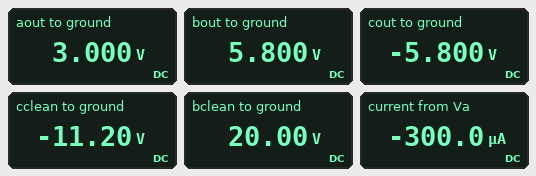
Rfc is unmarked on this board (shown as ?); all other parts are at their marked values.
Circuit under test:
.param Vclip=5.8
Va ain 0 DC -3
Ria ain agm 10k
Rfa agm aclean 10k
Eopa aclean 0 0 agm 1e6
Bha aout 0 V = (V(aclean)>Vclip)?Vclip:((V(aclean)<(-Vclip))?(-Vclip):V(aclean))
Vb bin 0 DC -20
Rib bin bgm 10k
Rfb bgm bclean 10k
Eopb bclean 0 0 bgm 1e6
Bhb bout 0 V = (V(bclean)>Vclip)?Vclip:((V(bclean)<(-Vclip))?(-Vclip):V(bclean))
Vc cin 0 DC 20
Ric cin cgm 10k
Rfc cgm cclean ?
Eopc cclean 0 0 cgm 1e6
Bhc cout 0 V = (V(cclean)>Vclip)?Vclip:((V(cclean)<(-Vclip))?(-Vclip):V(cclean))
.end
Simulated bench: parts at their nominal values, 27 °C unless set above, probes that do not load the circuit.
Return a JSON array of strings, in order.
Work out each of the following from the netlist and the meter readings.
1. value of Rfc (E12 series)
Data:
["5.6 kΩ"]
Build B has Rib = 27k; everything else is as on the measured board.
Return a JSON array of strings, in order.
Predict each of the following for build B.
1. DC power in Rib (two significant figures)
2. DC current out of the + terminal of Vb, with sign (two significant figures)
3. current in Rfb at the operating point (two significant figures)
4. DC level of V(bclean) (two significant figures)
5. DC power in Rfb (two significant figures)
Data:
["15 mW", "-740 µA", "740 µA", "7.4 V", "5.5 mW"]
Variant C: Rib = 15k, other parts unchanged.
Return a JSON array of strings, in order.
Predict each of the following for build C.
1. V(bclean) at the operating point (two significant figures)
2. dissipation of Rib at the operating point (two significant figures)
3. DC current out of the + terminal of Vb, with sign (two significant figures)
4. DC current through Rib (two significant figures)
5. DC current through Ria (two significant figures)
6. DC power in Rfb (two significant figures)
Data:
["13 V", "27 mW", "-1.3 mA", "1.3 mA", "300 µA", "18 mW"]
